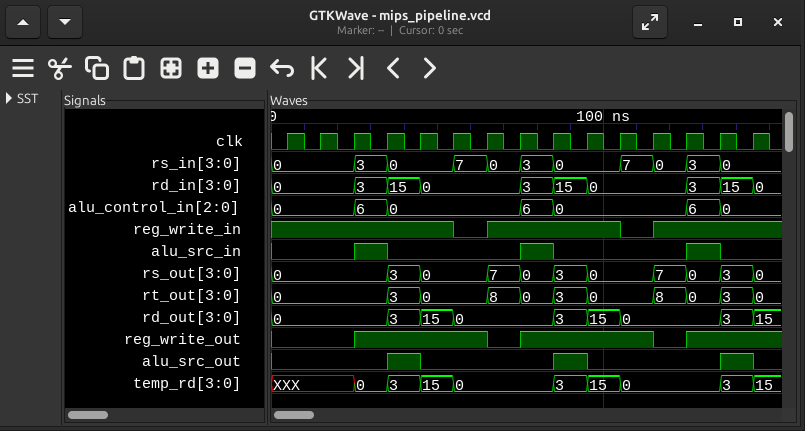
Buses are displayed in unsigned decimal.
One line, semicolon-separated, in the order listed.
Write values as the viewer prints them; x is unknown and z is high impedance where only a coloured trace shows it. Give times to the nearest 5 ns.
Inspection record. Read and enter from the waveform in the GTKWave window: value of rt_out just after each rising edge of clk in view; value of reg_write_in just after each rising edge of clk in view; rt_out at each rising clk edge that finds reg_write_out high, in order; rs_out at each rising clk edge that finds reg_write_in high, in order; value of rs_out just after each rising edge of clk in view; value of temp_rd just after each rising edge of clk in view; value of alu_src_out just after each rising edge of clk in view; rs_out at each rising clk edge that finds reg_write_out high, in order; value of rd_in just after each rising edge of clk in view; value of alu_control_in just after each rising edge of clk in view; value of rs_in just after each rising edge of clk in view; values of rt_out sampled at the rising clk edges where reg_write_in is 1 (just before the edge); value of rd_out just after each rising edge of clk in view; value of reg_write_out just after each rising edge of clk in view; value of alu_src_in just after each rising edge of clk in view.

0, 0, 0, 3, 0, 0, 8, 0, 3, 0, 0, 8, 0, 3, 0; 1 1 1 1 1 0 1 1 1 1 0 1 1 1 1; 0, 3, 0, 0, 0, 3, 0, 0, 0, 3; 0, 0, 0, 0, 3, 0, 7, 0, 3, 0, 7, 0, 3; 0, 0, 0, 3, 0, 0, 7, 0, 3, 0, 0, 7, 0, 3, 0; XXX, XXX, 0, 3, 15, 0, 0, 0, 3, 15, 0, 0, 0, 3, 15; 0 0 0 1 0 0 0 0 1 0 0 0 0 1 0; 0, 3, 0, 0, 0, 3, 0, 0, 0, 3; 0, 0, 3, 15, 0, 0, 0, 3, 15, 0, 0, 0, 3, 15, 0; 0, 0, 6, 0, 0, 0, 0, 6, 0, 0, 0, 0, 6, 0, 0; 0, 0, 3, 0, 0, 7, 0, 3, 0, 0, 7, 0, 3, 0, 0; 0, 0, 0, 0, 3, 0, 8, 0, 3, 0, 8, 0, 3; 0, 0, 0, 3, 15, 0, 0, 0, 3, 15, 0, 0, 0, 3, 15; 0 0 1 1 1 1 0 1 1 1 1 0 1 1 1; 0 0 1 0 0 0 0 1 0 0 0 0 1 0 0
